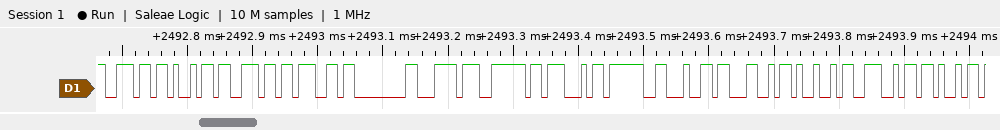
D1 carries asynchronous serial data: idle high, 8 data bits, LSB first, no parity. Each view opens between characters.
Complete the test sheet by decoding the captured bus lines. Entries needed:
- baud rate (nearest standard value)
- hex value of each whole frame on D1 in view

115200 baud
6E, 69, 6E, 67, 00, BC, 7E, 47, 3F, 64, 4C, 49, 4E, 4B
